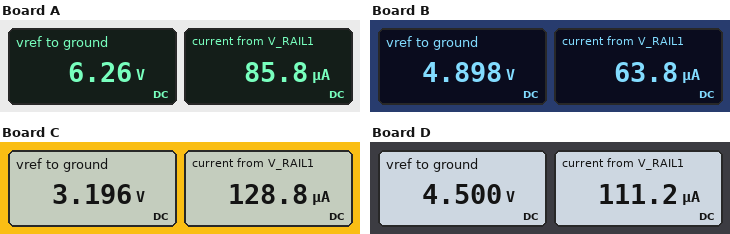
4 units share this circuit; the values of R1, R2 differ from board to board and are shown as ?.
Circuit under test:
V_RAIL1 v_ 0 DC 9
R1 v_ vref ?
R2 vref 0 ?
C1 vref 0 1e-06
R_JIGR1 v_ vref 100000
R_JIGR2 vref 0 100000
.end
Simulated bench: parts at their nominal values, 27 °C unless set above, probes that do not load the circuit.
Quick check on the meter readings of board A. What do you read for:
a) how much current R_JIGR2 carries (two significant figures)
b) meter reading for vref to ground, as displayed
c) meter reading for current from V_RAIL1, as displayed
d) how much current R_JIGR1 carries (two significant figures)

63 µA
6.26 V
85.8 µA
27 µA
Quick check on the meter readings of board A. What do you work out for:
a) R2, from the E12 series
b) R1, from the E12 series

270 kΩ
47 kΩ
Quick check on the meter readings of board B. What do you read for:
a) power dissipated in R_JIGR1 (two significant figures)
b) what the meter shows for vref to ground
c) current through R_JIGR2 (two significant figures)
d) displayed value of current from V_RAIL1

170 µW
4.898 V
49 µA
63.8 µA
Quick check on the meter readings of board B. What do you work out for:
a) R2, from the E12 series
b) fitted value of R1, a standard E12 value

330 kΩ
180 kΩ
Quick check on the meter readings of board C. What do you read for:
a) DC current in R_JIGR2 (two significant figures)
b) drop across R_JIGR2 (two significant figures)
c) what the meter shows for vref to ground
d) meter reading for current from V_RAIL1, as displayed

32 µA
3.2 V
3.196 V
128.8 µA
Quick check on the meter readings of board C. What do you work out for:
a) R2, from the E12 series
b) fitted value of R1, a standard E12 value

33 kΩ
82 kΩ
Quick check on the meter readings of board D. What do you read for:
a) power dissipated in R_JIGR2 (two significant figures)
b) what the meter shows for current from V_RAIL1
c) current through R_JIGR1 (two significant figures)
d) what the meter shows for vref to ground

200 µW
111.2 µA
45 µA
4.500 V
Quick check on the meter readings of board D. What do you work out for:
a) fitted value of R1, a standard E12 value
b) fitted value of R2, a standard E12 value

68 kΩ
68 kΩ
